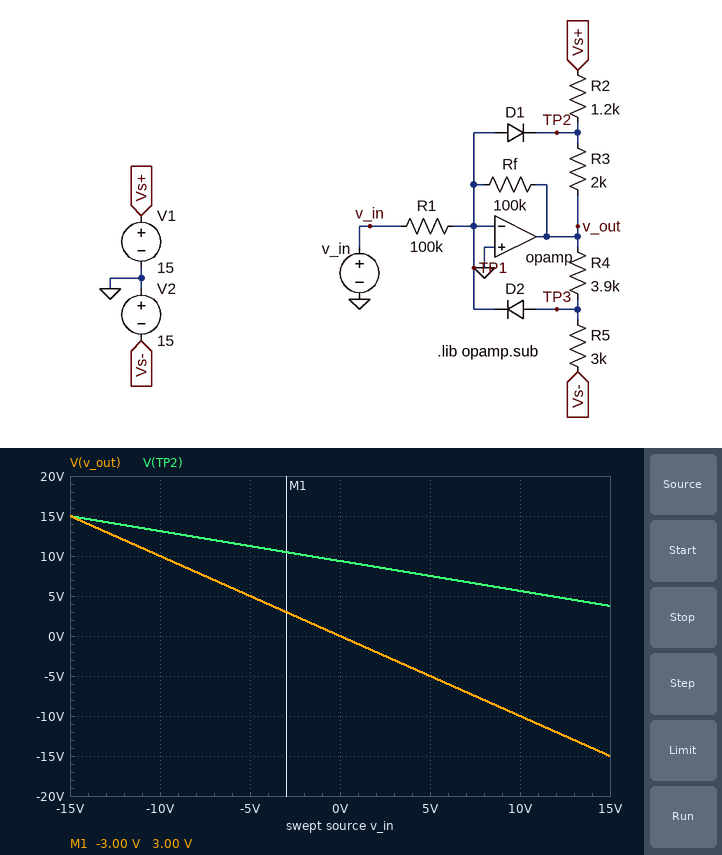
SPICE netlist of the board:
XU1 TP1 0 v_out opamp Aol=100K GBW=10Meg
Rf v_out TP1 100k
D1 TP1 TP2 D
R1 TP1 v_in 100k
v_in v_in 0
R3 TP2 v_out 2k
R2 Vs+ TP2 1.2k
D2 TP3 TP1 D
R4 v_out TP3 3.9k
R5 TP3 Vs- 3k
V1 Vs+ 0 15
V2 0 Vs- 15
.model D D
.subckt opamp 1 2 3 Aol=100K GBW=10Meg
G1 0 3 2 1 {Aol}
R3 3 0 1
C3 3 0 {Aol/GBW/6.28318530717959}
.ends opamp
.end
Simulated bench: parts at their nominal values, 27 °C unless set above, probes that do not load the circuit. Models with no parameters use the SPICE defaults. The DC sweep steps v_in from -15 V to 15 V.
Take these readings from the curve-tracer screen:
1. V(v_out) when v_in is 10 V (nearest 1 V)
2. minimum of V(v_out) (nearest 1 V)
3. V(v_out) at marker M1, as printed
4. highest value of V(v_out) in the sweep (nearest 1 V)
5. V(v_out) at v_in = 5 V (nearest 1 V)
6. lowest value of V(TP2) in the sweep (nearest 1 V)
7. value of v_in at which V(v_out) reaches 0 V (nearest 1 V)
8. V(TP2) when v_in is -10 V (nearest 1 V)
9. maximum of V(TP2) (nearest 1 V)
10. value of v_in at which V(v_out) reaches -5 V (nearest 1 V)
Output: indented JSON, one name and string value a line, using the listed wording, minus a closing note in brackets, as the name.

{
  "V(v_out) when v_in is 10 V": "-10 V",
  "minimum of V(v_out)": "-15 V",
  "V(v_out) at marker M1, as printed": "3.00 V",
  "highest value of V(v_out) in the sweep": "15 V",
  "V(v_out) at v_in = 5 V": "-5 V",
  "lowest value of V(TP2) in the sweep": "4 V",
  "value of v_in at which V(v_out) reaches 0 V": "0 V",
  "V(TP2) when v_in is -10 V": "13 V",
  "maximum of V(TP2)": "15 V",
  "value of v_in at which V(v_out) reaches -5 V": "5 V"
}
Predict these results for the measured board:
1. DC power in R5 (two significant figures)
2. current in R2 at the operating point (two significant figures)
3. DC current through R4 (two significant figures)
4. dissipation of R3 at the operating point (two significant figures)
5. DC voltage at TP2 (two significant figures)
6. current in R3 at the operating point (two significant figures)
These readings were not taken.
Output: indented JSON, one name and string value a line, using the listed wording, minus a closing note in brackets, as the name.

{
  "DC power in R5": "14 mW",
  "current in R2 at the operating point": "4.7 mA",
  "DC current through R4": "2.2 mA",
  "dissipation of R3 at the operating point": "44 mW",
  "DC voltage at TP2": "9.4 V",
  "current in R3 at the operating point": "4.7 mA"
}
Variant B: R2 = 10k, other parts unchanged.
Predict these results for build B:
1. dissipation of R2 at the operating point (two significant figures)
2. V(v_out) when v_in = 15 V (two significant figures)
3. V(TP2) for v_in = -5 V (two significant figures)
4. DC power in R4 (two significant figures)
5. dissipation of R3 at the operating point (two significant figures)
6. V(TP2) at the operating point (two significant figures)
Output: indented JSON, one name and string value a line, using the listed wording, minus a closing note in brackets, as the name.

{
  "dissipation of R2 at the operating point": "16 mW",
  "V(v_out) when v_in = 15 V": "-3.9 V",
  "V(TP2) for v_in = -5 V": "6.7 V",
  "DC power in R4": "18 mW",
  "dissipation of R3 at the operating point": "3.1 mW",
  "V(TP2) at the operating point": "2.5 V"
}
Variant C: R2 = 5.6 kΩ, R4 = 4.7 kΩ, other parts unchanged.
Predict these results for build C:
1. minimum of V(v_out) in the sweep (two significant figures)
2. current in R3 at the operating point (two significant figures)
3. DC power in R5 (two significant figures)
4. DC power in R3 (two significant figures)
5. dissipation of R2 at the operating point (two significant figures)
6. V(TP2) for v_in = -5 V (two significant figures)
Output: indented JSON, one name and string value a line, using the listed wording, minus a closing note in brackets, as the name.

{
  "minimum of V(v_out) in the sweep": "-6.3 V",
  "current in R3 at the operating point": "2.0 mA",
  "DC power in R5": "11 mW",
  "DC power in R3": "7.8 mW",
  "dissipation of R2 at the operating point": "22 mW",
  "V(TP2) for v_in = -5 V": "7.6 V"
}
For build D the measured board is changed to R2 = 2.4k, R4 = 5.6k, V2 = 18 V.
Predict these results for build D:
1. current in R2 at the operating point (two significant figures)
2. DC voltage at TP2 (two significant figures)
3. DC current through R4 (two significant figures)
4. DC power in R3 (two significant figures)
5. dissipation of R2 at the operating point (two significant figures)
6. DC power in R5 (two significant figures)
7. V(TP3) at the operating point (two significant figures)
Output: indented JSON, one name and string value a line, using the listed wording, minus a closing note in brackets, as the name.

{
  "current in R2 at the operating point": "3.4 mA",
  "DC voltage at TP2": "6.8 V",
  "DC current through R4": "2.1 mA",
  "DC power in R3": "23 mW",
  "dissipation of R2 at the operating point": "28 mW",
  "DC power in R5": "13 mW",
  "V(TP3) at the operating point": "-12 V"
}
